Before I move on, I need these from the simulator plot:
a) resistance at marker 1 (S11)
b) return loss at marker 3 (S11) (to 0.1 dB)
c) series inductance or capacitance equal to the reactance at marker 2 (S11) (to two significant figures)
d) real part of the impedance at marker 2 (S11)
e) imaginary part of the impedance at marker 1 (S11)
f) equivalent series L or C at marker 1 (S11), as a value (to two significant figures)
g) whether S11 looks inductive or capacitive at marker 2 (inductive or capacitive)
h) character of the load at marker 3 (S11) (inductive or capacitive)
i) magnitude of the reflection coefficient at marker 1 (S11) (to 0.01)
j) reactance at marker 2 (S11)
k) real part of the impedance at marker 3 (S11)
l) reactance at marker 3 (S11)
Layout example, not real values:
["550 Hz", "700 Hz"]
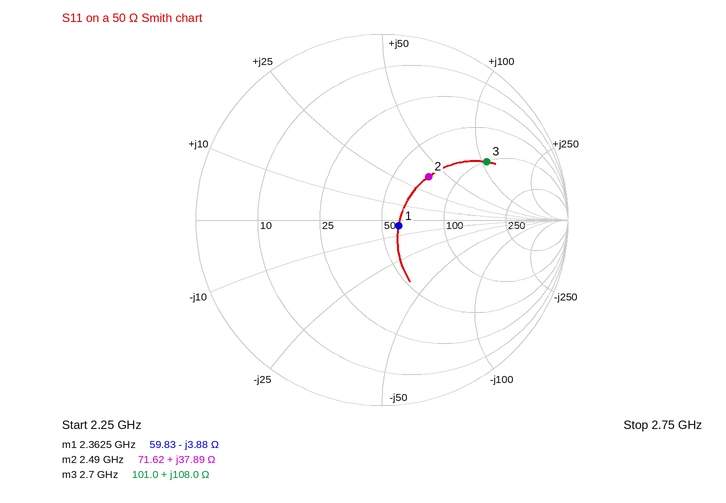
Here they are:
["59.83 Ω", "3.8 dB", "2.4 nH", "71.62 Ω", "-3.88 Ω", "17 pF", "inductive", "inductive", "0.10", "+37.89 Ω", "101.0 Ω", "+108.0 Ω"]
